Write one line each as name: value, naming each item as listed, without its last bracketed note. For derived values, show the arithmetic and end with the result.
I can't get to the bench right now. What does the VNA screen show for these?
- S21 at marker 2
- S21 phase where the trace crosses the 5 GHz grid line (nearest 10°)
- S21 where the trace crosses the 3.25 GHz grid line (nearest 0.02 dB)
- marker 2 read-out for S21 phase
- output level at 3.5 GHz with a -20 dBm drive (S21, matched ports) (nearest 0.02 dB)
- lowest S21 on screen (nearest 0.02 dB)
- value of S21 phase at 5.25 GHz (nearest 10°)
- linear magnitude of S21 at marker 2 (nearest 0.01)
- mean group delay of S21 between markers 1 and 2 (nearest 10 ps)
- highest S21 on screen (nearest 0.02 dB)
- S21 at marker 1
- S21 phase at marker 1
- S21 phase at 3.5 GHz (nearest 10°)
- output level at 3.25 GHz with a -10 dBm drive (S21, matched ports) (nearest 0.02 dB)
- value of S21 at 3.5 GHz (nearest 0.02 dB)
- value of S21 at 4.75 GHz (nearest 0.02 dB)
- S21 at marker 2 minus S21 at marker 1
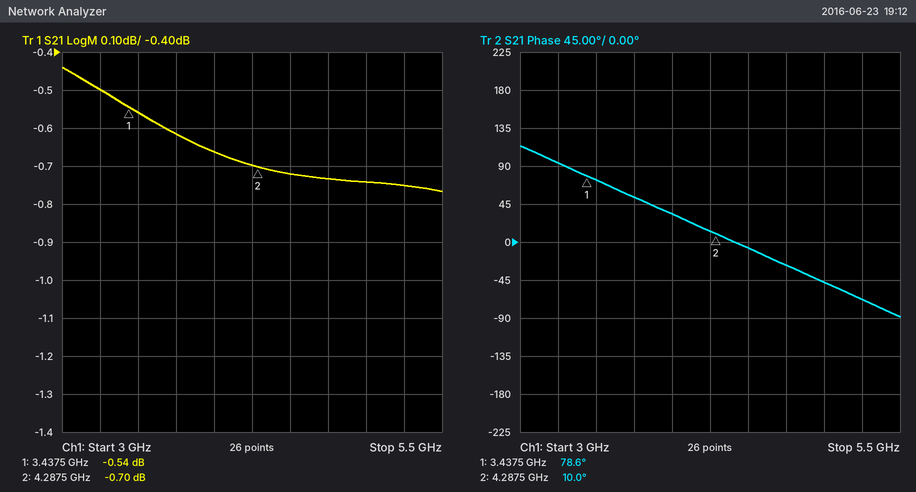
S21 at marker 2: -0.70 dB
S21 phase where the trace crosses the 5 GHz grid line: -50°
S21 where the trace crosses the 3.25 GHz grid line: -0.50 dB
marker 2 read-out for S21 phase: 10.0°
output level at 3.5 GHz with a -20 dBm drive (S21, matched ports): -20 dBm + (-0.56 dB) = -20.56 dBm
lowest S21 on screen: -0.76 dB
value of S21 phase at 5.25 GHz: -70°
linear magnitude of S21 at marker 2: 10^(-0.7/20) ≈ 0.92
mean group delay of S21 between markers 1 and 2: −(10° − (78.6°))/(360° × 850 MHz) ≈ 224 ps, so 220 ps to the nearest 10 ps
highest S21 on screen: -0.44 dB
S21 at marker 1: -0.54 dB
S21 phase at marker 1: 78.6°
S21 phase at 3.5 GHz: 70°
output level at 3.25 GHz with a -10 dBm drive (S21, matched ports): -10 dBm + (-0.50 dB) = -10.50 dBm
value of S21 at 3.5 GHz: -0.56 dB
value of S21 at 4.75 GHz: -0.74 dB
S21 at marker 2 minus S21 at marker 1: -0.7 − (-0.54) = -0.16 dB
